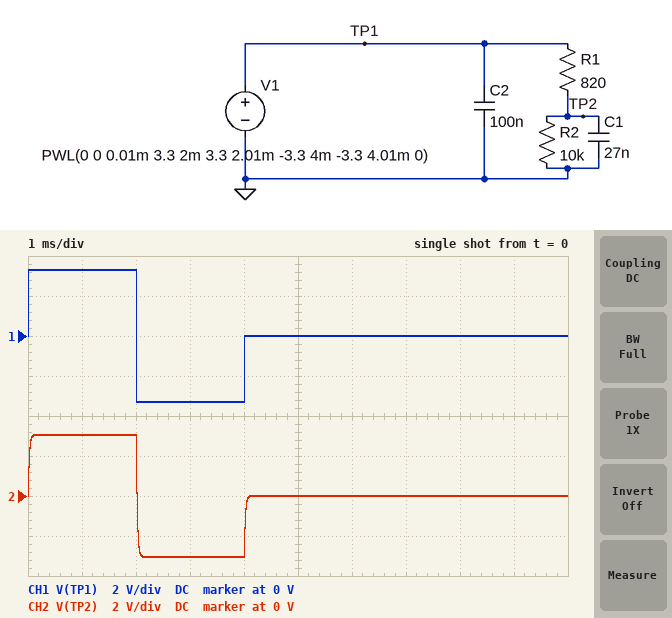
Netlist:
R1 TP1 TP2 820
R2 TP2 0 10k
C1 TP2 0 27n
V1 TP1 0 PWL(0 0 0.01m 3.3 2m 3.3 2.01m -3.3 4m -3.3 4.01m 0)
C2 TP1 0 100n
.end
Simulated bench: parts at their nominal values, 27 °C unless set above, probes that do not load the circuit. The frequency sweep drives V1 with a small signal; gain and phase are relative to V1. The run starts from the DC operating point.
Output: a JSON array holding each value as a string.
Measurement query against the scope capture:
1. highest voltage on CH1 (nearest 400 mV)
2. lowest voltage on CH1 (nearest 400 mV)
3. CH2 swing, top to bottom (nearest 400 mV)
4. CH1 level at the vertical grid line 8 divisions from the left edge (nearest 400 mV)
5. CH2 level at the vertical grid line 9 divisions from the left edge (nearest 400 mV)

["3.2 V", "-3.2 V", "6.0 V", "0 V", "0 V"]
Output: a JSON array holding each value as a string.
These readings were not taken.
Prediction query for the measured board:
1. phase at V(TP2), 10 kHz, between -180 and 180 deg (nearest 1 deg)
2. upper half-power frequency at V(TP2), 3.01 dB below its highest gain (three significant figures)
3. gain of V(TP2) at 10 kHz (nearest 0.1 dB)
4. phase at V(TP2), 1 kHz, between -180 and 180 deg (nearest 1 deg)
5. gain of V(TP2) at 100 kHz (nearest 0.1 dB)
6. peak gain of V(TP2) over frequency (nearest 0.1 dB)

["-52 deg", "7.78 kHz", "-4.9 dB", "-7 deg", "-22.9 dB", "-0.7 dB"]
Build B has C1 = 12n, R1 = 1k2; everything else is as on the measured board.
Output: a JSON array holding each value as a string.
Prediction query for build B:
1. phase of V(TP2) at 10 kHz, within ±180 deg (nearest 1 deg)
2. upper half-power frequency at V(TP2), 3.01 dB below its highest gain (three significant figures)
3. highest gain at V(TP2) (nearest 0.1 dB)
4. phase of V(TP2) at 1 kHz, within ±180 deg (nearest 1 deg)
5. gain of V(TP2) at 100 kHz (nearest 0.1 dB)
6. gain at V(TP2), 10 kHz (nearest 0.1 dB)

["-39 deg", "12.4 kHz", "-1.0 dB", "-5 deg", "-19.2 dB", "-3.2 dB"]
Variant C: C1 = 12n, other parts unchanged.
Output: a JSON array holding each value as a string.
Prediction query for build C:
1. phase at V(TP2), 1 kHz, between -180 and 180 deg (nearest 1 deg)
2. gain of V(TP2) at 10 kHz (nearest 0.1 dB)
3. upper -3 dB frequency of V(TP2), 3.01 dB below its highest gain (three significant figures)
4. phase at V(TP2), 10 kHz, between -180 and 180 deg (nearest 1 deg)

["-3 deg", "-1.9 dB", "17.5 kHz", "-30 deg"]
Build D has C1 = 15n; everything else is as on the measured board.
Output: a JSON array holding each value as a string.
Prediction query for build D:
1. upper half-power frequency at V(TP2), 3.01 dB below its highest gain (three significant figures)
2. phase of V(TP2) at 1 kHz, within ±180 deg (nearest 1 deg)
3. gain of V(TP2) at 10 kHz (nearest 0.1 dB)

["14.0 kHz", "-4 deg", "-2.5 dB"]
